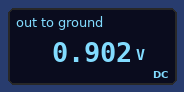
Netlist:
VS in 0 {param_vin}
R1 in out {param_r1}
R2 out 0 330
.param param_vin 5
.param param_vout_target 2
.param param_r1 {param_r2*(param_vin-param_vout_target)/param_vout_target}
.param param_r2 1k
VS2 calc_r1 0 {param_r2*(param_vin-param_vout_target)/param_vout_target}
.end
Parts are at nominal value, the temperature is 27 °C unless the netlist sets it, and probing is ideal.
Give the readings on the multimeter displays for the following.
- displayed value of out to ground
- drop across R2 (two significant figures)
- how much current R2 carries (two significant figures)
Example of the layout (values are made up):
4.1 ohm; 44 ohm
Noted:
0.902 V; 900 mV; 2.7 mA
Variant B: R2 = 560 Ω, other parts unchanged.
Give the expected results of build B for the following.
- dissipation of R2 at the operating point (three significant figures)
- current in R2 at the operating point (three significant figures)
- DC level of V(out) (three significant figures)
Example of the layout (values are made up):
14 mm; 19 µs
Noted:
3.30 mW; 2.43 mA; 1.36 V
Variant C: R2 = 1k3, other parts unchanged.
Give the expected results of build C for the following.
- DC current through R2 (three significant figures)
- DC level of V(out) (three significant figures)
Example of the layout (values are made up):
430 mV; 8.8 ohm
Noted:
1.79 mA; 2.32 V
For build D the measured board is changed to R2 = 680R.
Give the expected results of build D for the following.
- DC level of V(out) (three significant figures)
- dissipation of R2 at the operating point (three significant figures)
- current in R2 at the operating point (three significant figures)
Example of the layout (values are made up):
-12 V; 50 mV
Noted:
1.56 V; 3.58 mW; 2.29 mA
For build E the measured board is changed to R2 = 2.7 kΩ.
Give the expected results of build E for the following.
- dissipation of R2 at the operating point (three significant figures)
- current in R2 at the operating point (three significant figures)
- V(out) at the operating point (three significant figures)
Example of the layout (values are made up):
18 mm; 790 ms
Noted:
3.83 mW; 1.19 mA; 3.21 V
